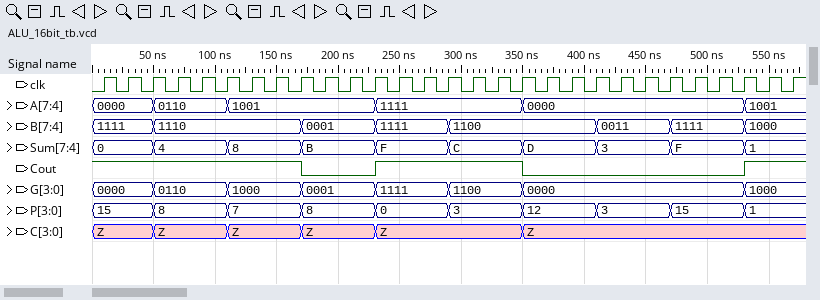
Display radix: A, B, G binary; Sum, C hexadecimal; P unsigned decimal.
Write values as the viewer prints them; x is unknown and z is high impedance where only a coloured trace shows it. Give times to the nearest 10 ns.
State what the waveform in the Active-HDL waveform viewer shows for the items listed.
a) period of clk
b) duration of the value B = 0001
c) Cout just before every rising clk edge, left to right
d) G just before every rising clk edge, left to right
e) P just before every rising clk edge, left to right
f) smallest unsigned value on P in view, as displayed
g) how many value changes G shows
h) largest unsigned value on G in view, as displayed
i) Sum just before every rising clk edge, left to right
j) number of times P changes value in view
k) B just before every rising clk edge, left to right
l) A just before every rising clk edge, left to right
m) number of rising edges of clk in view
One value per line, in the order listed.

20 ns
60 ns
1 1 1 1 1 1 1 1 1 0 0 0 1 1 1 1 1 1 0 0 0 0 0 0 0 0 0 1 1
0000, 0000, 0000, 0110, 0110, 0110, 1000, 1000, 1000, 0001, 0001, 0001, 1111, 1111, 1111, 1100, 1100, 1100, 0000, 0000, 0000, 0000, 0000, 0000, 0000, 0000, 0000, 1000, 1000
15, 15, 15, 8, 8, 8, 7, 7, 7, 8, 8, 8, 0, 0, 0, 3, 3, 3, 12, 12, 12, 3, 3, 3, 15, 15, 15, 1, 1
0
7
1111
0, 0, 0, 4, 4, 4, 8, 8, 8, B, B, B, F, F, F, C, C, C, D, D, D, 3, 3, 3, F, F, F, 1, 1
9
1111, 1111, 1111, 1110, 1110, 1110, 1110, 1110, 1110, 0001, 0001, 0001, 1111, 1111, 1111, 1100, 1100, 1100, 1100, 1100, 1100, 0011, 0011, 0011, 1111, 1111, 1111, 1000, 1000
0000, 0000, 0000, 0110, 0110, 0110, 1001, 1001, 1001, 1001, 1001, 1001, 1111, 1111, 1111, 1111, 1111, 1111, 0000, 0000, 0000, 0000, 0000, 0000, 0000, 0000, 0000, 1001, 1001
29
